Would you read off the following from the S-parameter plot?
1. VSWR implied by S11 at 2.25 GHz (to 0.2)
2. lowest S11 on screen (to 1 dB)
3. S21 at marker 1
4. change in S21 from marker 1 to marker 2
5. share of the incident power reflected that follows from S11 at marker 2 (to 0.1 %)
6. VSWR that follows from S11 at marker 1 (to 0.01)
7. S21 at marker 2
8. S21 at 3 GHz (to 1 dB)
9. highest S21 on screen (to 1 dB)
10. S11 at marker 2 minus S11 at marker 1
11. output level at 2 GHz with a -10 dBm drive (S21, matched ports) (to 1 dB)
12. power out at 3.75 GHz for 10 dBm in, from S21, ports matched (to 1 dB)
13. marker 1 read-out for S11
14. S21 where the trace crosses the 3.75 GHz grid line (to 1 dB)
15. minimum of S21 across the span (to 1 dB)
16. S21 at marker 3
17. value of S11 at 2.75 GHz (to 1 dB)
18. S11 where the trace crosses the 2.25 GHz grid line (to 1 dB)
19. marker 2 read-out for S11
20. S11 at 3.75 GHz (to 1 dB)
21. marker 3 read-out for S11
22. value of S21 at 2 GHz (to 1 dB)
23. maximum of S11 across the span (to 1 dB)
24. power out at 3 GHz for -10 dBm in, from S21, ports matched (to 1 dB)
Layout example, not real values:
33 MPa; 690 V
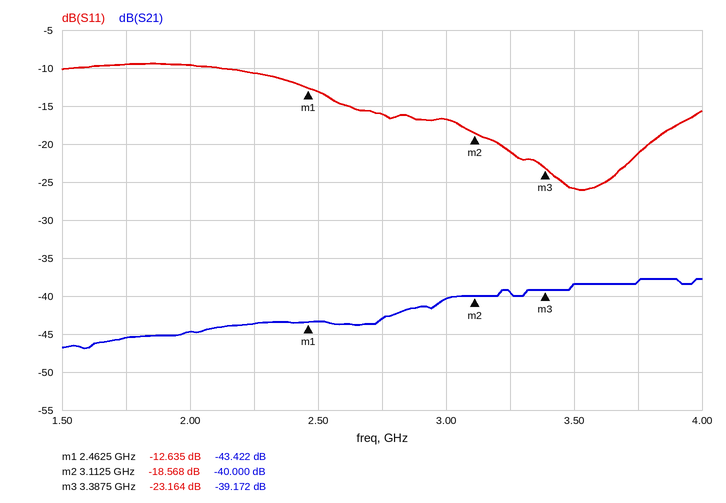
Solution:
1.8; -26 dB; -43.422 dB; 3.422 dB; 1.4 %; 1.61; -40.000 dB; -40 dB; -38 dB; -5.933 dB; -55 dBm; -28 dBm; -12.635 dB; -38 dB; -47 dB; -39.172 dB; -16 dB; -11 dB; -18.568 dB; -21 dB; -23.164 dB; -45 dB; -9 dB; -50 dBm
